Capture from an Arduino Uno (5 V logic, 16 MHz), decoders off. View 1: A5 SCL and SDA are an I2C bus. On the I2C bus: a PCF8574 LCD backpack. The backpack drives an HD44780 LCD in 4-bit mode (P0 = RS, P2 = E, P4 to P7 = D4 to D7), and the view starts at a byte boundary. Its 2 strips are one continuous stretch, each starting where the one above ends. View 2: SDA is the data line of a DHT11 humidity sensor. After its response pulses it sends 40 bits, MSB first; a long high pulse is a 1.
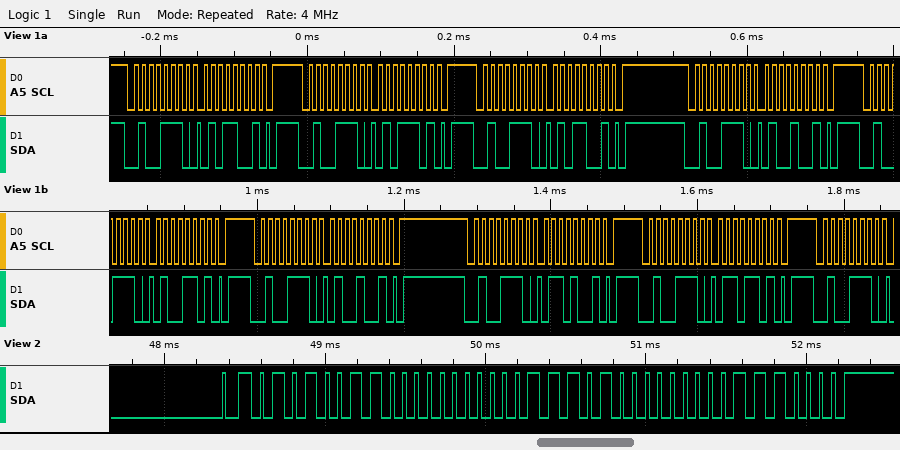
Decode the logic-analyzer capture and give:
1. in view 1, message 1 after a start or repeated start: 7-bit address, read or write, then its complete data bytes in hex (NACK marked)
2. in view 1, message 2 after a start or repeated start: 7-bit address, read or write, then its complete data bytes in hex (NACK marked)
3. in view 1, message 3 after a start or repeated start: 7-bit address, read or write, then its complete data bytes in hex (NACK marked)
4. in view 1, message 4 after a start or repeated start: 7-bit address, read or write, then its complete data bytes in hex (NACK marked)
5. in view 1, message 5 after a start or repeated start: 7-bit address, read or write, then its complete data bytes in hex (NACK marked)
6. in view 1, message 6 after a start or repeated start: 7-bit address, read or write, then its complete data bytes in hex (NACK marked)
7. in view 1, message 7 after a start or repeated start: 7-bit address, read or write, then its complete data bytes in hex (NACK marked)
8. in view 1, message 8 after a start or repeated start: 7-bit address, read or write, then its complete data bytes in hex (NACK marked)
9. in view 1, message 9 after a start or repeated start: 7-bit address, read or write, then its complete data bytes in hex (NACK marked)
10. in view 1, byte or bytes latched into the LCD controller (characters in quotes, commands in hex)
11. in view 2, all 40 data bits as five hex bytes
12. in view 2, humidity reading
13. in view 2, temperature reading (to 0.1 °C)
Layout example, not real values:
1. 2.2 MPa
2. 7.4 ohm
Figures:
1. 0x27 write: 59
2. 0x27 write: 5D
3. 0x27 write: 59
4. 0x27 write: 49
5. 0x27 write: 4D
6. 0x27 write: 49
7. 0x27 write: 69
8. 0x27 write: 6D
9. 0x27 write
10. 'T'
11. 53 00 1D 00 70
12. 83 %
13. 29.0 °C
